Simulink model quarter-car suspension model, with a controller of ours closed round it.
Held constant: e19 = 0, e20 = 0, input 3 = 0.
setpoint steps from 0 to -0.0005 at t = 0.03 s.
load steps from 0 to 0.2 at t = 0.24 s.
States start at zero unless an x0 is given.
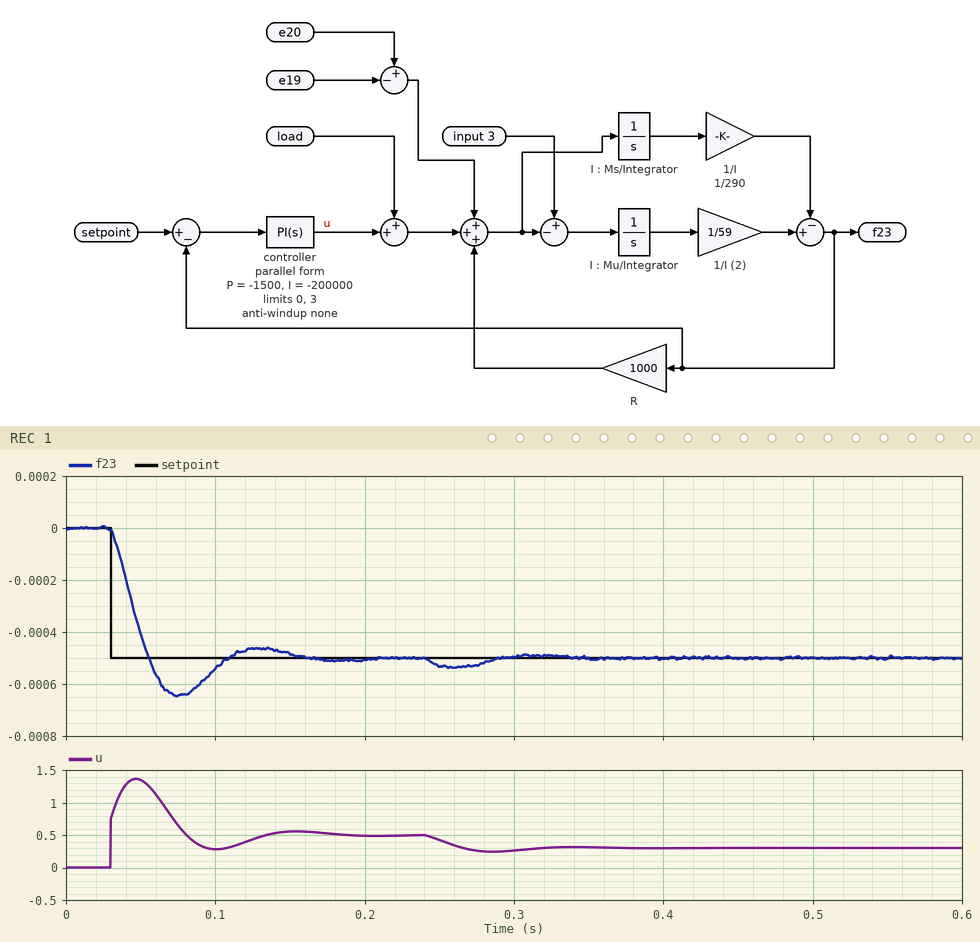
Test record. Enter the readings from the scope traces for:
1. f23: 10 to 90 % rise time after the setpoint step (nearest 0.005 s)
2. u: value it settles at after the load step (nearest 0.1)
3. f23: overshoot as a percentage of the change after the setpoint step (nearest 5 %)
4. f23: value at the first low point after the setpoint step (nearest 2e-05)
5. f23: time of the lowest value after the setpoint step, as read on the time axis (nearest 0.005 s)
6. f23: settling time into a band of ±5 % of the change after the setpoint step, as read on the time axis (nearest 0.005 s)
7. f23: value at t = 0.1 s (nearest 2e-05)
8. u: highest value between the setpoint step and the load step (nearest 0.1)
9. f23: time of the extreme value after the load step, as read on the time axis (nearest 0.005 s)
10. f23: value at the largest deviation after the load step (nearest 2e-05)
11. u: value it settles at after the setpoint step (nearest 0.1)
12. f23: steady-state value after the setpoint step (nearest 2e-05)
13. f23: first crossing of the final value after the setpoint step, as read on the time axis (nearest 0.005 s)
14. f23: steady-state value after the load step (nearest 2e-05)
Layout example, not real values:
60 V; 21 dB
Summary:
0.020 s; 0.3; 30 %; -0.00064; 0.075 s; 0.145 s; -0.00054; 1.4; 0.260 s; -0.00054; 0.5; -0.00050; 0.055 s; -0.00050
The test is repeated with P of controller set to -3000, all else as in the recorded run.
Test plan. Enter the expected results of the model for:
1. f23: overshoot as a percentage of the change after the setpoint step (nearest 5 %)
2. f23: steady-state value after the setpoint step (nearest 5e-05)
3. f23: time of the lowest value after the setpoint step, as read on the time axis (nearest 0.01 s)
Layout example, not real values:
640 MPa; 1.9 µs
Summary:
15 %; -0.00050; 0.07 s
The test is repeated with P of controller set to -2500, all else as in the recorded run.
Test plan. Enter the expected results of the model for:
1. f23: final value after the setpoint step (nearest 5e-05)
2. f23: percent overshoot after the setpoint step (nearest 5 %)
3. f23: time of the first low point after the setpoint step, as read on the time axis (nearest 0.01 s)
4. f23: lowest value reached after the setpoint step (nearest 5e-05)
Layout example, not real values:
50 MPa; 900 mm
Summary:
-0.00050; 20 %; 0.07 s; -0.00060
